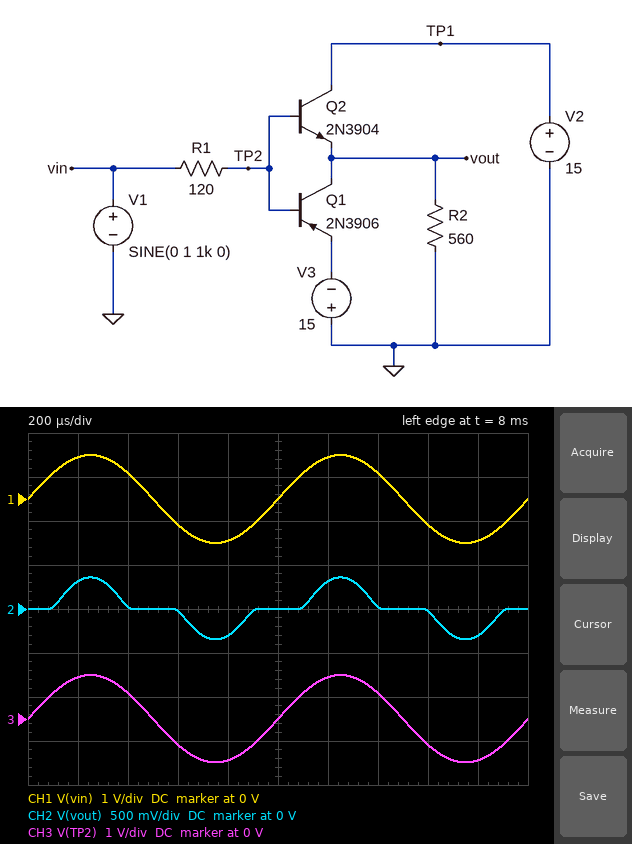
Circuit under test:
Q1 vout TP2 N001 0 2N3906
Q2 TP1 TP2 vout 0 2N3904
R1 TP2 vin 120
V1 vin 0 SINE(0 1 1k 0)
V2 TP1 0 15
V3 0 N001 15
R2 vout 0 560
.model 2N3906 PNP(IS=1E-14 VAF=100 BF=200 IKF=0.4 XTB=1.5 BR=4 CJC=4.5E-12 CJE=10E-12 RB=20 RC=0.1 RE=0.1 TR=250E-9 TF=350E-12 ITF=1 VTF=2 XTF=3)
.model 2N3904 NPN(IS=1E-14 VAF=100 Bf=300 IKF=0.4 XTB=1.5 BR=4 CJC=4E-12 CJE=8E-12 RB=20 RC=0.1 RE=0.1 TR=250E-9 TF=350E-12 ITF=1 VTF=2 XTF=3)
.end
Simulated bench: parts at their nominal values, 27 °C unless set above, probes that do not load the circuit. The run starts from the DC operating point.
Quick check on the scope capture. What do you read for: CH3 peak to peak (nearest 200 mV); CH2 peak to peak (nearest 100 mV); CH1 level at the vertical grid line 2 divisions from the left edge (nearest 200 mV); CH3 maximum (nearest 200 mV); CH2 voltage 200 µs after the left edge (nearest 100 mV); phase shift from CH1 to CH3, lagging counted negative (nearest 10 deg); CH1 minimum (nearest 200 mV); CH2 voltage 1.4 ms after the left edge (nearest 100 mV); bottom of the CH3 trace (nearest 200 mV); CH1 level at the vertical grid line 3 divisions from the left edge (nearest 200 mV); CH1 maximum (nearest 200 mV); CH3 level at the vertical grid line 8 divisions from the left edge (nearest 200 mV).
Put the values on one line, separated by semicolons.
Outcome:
2.0 V; 700 mV; 600 mV; 1.0 V; 300 mV; 0 deg; -1.0 V; 0 V; -1.0 V; -600 mV; 1.0 V; -600 mV
